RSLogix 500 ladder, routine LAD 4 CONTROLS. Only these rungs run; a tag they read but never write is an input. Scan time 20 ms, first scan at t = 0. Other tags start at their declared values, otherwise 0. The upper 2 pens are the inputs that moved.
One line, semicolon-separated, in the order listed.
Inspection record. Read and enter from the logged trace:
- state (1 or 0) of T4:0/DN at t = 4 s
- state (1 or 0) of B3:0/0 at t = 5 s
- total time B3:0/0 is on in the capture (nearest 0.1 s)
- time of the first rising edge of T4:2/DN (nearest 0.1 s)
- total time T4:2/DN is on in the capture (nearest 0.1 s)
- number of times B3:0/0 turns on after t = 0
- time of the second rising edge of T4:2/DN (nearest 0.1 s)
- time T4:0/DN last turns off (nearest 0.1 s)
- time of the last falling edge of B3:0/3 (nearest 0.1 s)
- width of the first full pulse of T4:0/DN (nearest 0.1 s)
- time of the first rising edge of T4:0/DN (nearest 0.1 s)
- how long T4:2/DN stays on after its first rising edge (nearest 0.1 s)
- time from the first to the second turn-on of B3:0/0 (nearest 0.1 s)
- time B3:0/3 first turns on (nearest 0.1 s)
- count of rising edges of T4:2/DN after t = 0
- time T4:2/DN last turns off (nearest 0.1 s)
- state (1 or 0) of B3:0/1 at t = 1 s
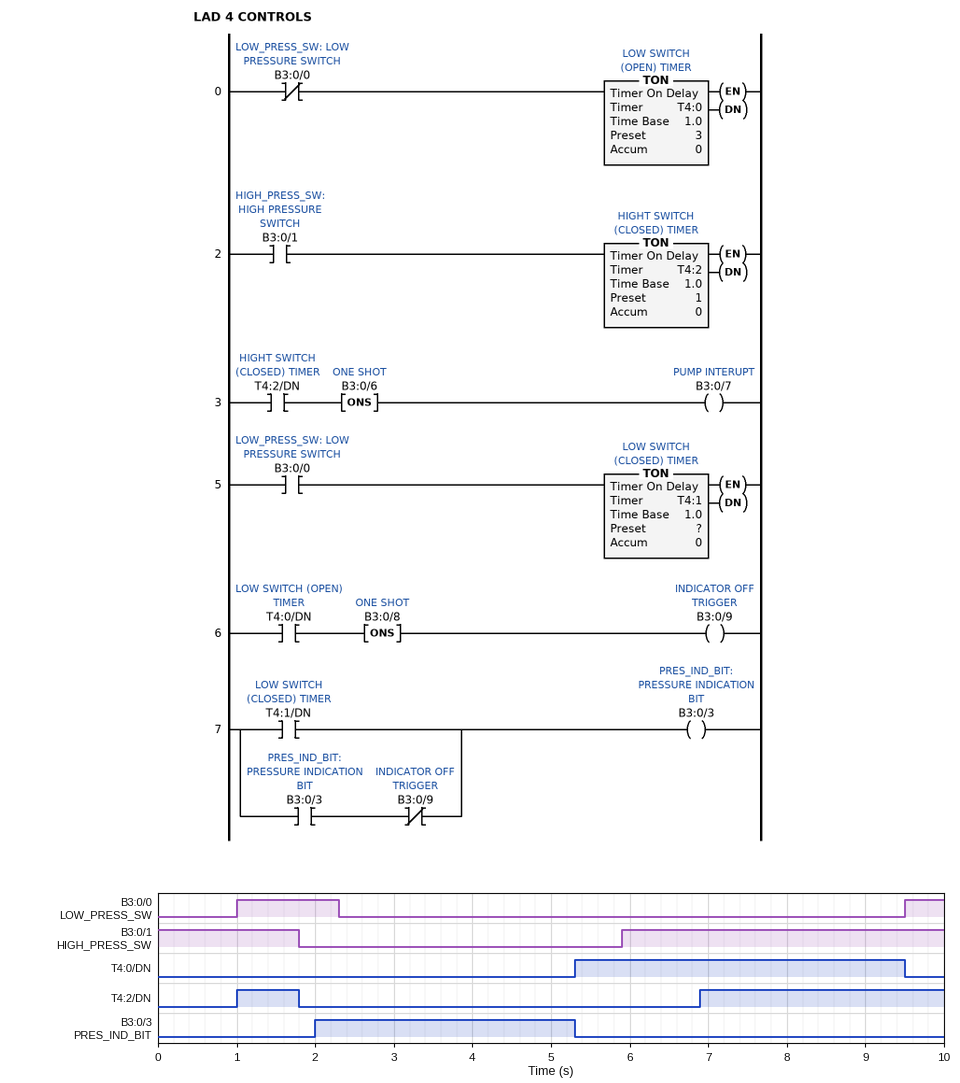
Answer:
0; 0; 1.8 s; 1.0 s; 3.9 s; 2; 6.9 s; 9.5 s; 5.3 s; 4.2 s; 5.3 s; 0.8 s; 8.5 s; 2.0 s; 2; 1.8 s; 1
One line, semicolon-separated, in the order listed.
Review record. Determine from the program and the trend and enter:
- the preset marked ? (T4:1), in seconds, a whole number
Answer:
1 s
